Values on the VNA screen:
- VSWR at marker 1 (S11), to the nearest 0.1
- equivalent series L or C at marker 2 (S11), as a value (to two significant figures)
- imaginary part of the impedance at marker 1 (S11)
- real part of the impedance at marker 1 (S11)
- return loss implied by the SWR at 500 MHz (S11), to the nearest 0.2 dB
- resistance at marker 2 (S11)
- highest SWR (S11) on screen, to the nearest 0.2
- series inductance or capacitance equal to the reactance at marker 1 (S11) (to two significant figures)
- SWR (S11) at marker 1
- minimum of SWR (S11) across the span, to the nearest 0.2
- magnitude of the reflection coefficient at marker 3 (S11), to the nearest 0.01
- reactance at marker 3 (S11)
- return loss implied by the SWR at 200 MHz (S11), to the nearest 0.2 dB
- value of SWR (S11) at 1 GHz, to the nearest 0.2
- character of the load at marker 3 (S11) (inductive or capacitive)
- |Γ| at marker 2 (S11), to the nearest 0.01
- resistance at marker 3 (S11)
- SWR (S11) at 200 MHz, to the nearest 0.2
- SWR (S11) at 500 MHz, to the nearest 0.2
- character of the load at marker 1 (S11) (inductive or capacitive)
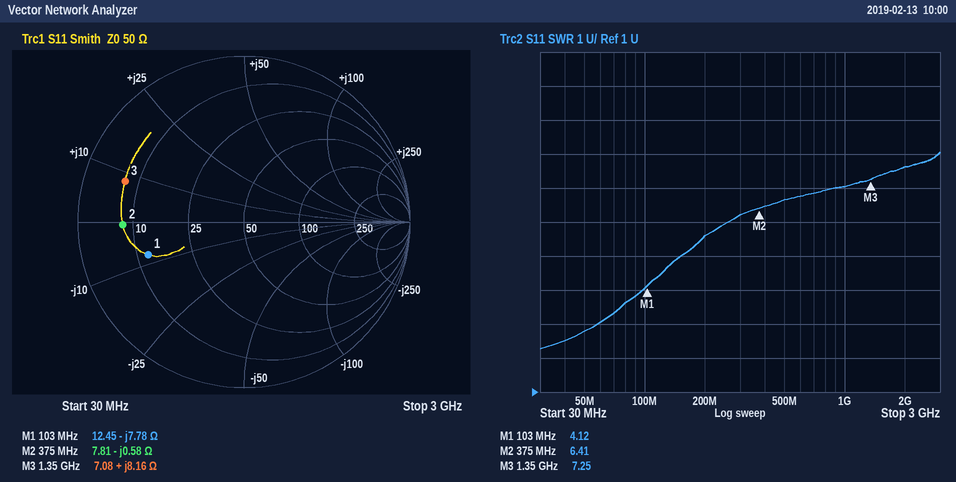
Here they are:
4.1
730 pF
-7.78 Ω
12.45 Ω
2.6 dB
7.81 Ω
8.0
200 pF
4.12
2.2
0.76
+8.16 Ω
3.2 dB
7.0
inductive
0.73
7.08 Ω
5.6
6.6
capacitive
